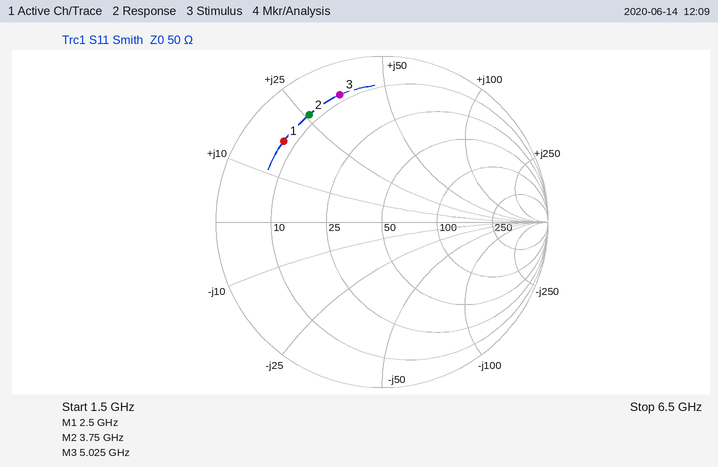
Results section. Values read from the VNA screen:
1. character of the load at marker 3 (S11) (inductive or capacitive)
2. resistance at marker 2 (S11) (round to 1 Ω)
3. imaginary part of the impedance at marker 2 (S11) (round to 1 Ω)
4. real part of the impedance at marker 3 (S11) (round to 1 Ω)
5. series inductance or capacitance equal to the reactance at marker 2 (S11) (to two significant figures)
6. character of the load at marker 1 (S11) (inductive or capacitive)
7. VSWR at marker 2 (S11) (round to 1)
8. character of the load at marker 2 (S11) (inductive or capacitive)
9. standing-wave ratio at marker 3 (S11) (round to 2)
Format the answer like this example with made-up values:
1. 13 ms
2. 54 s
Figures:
1. inductive
2. 8 Ω
3. +26 Ω
4. 8 Ω
5. 1.1 nH
6. inductive
7. 8
8. inductive
9. 10
